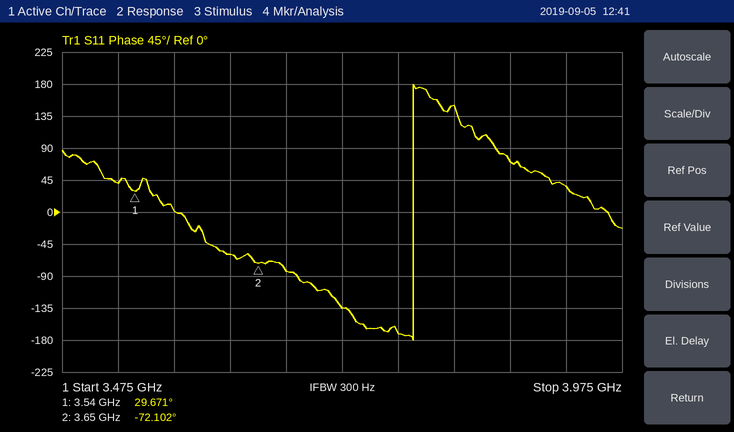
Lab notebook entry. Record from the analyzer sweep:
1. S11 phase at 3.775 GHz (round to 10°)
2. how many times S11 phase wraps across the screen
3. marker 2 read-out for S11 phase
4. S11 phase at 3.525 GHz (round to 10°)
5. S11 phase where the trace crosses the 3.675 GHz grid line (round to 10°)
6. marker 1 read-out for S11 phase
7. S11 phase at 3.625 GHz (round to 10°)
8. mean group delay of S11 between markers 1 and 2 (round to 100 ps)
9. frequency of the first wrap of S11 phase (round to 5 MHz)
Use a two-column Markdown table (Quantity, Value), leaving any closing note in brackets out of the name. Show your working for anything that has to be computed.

| Quantity | Value |
|---|---|
| S11 phase at 3.775 GHz | -170° |
| how many times S11 phase wraps across the screen | 1 |
| marker 2 read-out for S11 phase | -72.102° |
| S11 phase at 3.525 GHz | 40° |
| S11 phase where the trace crosses the 3.675 GHz grid line | -80° |
| marker 1 read-out for S11 phase | 29.671° |
| S11 phase at 3.625 GHz | -60° |
| mean group delay of S11 between markers 1 and 2 | −(-72.102° − (29.671°))/(360° × 110 MHz) ≈ 2.6 ns |
| frequency of the first wrap of S11 phase | 3.790 GHz |
